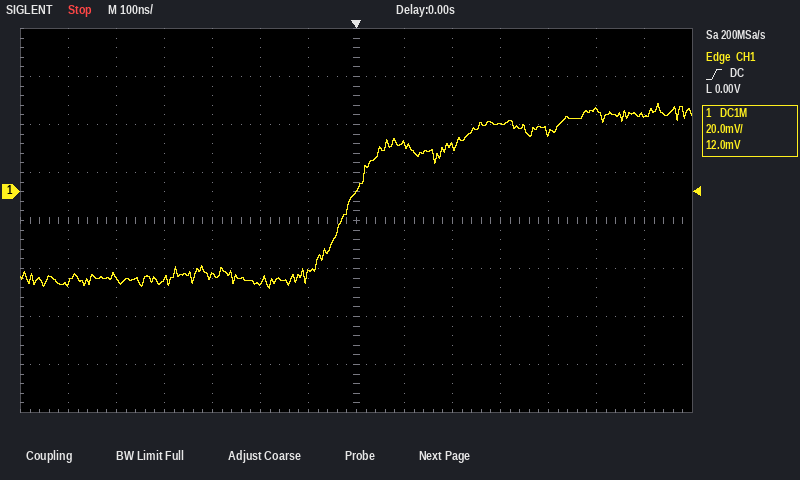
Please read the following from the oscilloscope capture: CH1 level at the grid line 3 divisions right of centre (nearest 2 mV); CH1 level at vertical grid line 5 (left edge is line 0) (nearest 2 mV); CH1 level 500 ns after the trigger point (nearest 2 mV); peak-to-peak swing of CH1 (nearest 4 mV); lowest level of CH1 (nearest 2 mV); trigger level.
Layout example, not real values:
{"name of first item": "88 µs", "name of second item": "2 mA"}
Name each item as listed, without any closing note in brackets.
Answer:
{"CH1 level at the grid line 3 divisions right of centre": "28 mV", "CH1 level at vertical grid line 5 (left edge is line 0)": "-38 mV", "CH1 level 500 ns after the trigger point": "34 mV", "peak-to-peak swing of CH1": "76 mV", "lowest level of CH1": "-40 mV", "trigger level": "0.00 V"}
